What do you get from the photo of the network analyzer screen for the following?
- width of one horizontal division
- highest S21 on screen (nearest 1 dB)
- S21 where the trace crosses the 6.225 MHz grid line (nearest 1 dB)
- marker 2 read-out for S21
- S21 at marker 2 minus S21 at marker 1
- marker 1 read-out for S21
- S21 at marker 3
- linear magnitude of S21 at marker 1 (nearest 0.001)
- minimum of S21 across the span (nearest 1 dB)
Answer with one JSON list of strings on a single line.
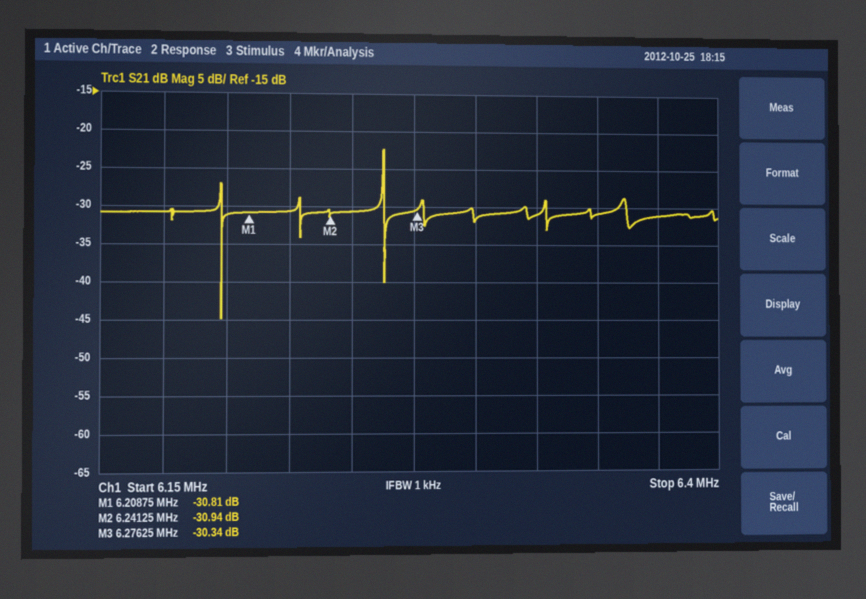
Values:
["25 kHz", "-22 dB", "-31 dB", "-30.94 dB", "-0.13 dB", "-30.81 dB", "-30.34 dB", "0.029", "-45 dB"]
